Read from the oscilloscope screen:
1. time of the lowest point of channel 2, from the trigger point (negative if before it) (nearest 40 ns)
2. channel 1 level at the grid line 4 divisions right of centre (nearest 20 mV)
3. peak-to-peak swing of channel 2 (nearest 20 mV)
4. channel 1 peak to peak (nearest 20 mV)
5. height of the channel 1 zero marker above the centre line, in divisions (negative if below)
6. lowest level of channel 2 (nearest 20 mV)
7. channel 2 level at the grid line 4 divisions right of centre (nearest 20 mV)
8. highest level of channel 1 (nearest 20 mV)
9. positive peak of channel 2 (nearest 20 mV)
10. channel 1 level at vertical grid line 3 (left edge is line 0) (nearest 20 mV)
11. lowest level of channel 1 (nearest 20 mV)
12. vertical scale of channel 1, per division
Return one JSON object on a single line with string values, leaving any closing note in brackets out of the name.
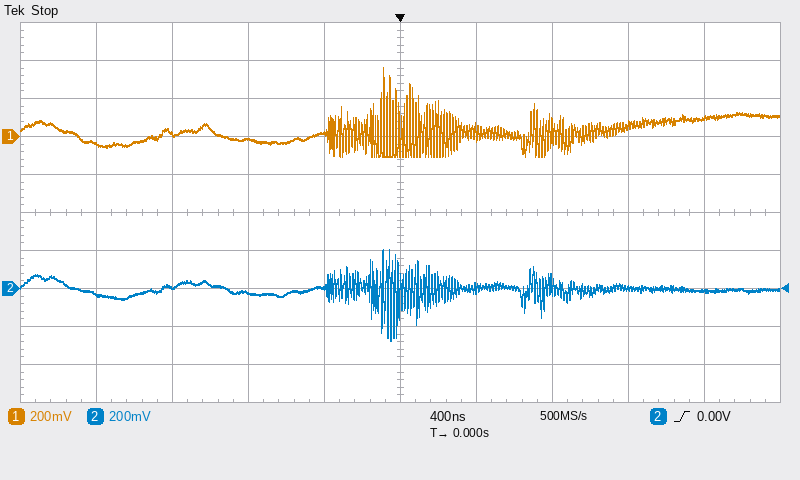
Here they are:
{"time of the lowest point of channel 2, from the trigger point (negative if before it)": "-40 ns", "channel 1 level at the grid line 4 divisions right of centre": "100 mV", "peak-to-peak swing of channel 2": "480 mV", "channel 1 peak to peak": "460 mV", "height of the channel 1 zero marker above the centre line, in divisions": "+2.0 div", "lowest level of channel 2": "-280 mV", "channel 2 level at the grid line 4 divisions right of centre": "-20 mV", "highest level of channel 1": "360 mV", "positive peak of channel 2": "200 mV", "channel 1 level at vertical grid line 3 (left edge is line 0)": "-20 mV", "lowest level of channel 1": "-100 mV", "vertical scale of channel 1, per division": "200 mV"}
